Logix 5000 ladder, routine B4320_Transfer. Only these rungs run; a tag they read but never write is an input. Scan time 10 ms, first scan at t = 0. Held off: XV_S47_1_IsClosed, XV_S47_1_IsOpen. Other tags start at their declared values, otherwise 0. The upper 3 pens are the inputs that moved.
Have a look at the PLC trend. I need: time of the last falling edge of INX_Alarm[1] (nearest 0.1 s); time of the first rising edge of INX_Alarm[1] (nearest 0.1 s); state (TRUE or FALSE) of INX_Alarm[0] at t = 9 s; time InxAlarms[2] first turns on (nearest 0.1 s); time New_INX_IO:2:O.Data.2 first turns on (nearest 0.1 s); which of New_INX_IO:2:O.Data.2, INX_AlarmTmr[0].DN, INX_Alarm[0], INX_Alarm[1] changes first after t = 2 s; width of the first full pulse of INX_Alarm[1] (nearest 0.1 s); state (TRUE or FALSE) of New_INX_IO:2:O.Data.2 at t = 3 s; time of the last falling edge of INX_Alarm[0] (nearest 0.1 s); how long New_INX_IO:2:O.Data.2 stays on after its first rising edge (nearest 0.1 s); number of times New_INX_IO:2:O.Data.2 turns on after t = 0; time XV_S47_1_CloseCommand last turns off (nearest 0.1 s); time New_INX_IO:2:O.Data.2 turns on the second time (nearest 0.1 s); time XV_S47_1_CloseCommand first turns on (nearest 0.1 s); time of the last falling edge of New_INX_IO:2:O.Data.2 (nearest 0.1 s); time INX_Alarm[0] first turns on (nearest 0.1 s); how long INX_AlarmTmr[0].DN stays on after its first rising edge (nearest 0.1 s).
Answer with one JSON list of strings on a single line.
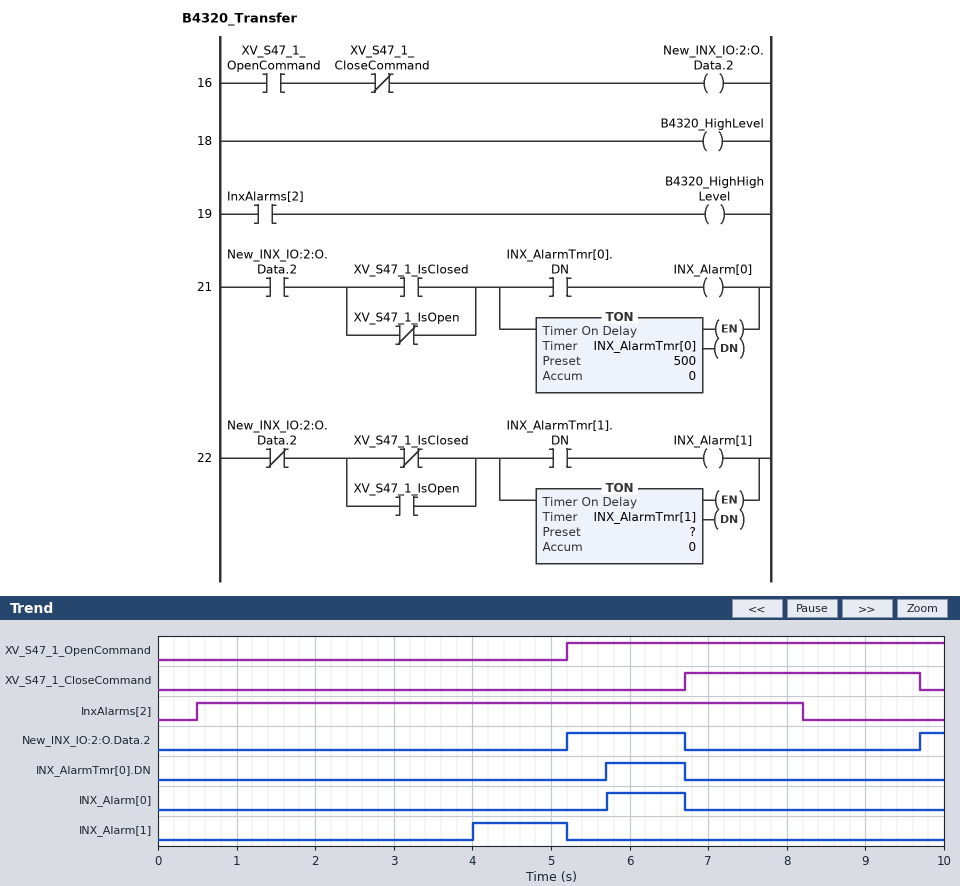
["5.2 s", "4.0 s", "FALSE", "0.5 s", "5.2 s", "INX_Alarm[1]", "1.2 s", "FALSE", "6.7 s", "1.5 s", "2", "9.7 s", "9.7 s", "6.7 s", "6.7 s", "5.7 s", "1.0 s"]
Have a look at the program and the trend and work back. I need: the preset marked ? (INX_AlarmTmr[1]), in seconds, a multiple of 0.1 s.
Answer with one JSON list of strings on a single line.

["4.0 s"]
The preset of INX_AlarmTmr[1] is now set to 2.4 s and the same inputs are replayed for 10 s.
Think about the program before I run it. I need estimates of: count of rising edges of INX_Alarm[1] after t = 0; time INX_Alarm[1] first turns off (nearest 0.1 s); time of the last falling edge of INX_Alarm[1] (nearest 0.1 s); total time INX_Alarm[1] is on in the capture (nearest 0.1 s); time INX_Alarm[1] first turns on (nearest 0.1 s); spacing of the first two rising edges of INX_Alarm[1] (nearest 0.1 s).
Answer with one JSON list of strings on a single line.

["2", "5.2 s", "9.7 s", "3.4 s", "2.4 s", "6.7 s"]
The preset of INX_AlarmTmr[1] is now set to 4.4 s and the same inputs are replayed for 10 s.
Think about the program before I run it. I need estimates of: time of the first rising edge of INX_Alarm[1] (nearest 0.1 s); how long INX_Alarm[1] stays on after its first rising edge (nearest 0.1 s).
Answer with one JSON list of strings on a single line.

["4.4 s", "0.8 s"]
